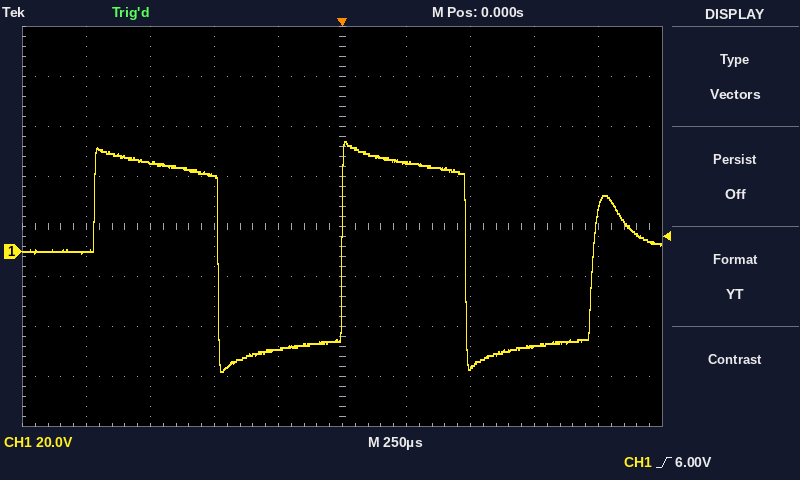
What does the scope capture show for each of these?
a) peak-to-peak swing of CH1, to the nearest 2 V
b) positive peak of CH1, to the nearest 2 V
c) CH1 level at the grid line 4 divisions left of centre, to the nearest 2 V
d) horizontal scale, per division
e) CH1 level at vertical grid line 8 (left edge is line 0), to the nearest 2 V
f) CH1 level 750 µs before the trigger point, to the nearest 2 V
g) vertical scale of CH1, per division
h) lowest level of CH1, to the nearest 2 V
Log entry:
92 V
44 V
0 V
250 µs
-38 V
36 V
20 V
-48 V
